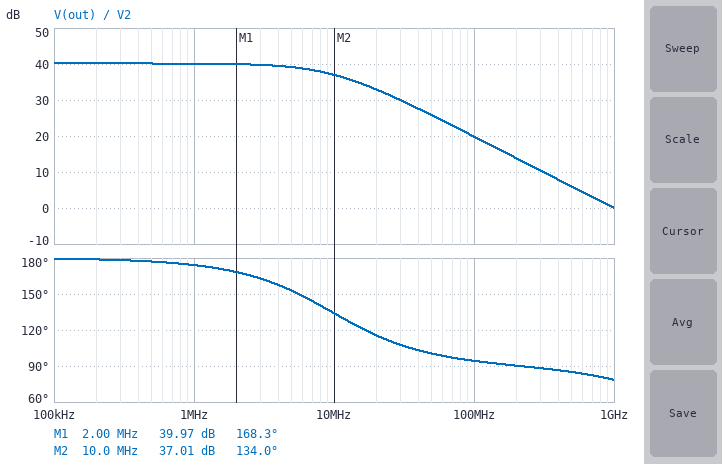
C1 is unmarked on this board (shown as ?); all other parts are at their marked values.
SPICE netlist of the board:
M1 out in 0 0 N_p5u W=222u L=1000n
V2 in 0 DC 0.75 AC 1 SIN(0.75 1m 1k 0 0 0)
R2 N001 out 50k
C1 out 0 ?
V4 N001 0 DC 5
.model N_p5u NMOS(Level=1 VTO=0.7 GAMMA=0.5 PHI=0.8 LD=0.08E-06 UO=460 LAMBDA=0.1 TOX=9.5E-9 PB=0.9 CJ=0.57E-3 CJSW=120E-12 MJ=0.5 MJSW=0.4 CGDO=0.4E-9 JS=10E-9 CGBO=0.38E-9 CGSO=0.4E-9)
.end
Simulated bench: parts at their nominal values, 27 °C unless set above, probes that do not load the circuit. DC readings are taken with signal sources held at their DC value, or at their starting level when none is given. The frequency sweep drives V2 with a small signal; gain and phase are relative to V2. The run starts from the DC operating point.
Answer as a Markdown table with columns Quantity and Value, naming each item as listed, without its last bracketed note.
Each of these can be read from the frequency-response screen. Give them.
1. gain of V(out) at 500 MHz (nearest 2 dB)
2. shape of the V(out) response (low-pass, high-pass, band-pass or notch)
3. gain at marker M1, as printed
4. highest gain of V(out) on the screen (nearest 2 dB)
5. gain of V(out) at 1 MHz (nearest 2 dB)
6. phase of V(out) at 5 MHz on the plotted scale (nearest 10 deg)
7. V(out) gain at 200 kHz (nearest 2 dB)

| Quantity | Value |
|---|---|
| gain of V(out) at 500 MHz | 6 dB |
| shape of the V(out) response | low-pass |
| gain at marker M1, as printed | 39.97 dB |
| highest gain of V(out) on the screen | 40 dB |
| gain of V(out) at 1 MHz | 40 dB |
| phase of V(out) at 5 MHz on the plotted scale | 150 deg |
| V(out) gain at 200 kHz | 40 dB |
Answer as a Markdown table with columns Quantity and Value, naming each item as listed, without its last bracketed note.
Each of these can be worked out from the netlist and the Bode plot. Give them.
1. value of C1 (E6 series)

| Quantity | Value |
|---|---|
| value of C1 | 330 fF |
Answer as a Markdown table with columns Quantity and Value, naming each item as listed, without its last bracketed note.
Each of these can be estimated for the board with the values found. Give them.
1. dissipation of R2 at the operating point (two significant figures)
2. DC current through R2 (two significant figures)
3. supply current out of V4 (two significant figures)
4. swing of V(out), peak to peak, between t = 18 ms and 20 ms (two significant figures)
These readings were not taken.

| Quantity | Value |
|---|---|
| dissipation of R2 at the operating point | 210 µW |
| DC current through R2 | 65 µA |
| supply current out of V4 | 65 µA |
| swing of V(out), peak to peak, between t = 18 ms and 20 ms | 200 mV |
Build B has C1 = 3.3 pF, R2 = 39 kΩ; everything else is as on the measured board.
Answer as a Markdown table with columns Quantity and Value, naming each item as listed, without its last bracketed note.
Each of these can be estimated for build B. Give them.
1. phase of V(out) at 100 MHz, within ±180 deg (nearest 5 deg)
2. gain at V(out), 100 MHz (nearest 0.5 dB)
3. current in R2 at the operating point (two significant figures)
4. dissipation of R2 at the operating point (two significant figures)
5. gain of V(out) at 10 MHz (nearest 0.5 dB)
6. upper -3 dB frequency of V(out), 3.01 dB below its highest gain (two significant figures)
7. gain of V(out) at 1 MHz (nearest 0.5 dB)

| Quantity | Value |
|---|---|
| phase of V(out) at 100 MHz, within ±180 deg | 90 deg |
| gain at V(out), 100 MHz | 2.0 dB |
| current in R2 at the operating point | 68 µA |
| dissipation of R2 at the operating point | 180 µW |
| gain of V(out) at 10 MHz | 22.0 dB |
| upper -3 dB frequency of V(out), 3.01 dB below its highest gain | 1.5 MHz |
| gain of V(out) at 1 MHz | 37.0 dB |
